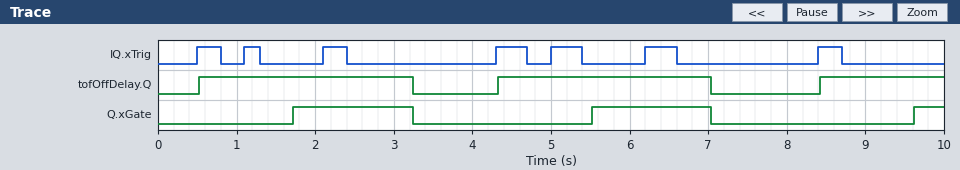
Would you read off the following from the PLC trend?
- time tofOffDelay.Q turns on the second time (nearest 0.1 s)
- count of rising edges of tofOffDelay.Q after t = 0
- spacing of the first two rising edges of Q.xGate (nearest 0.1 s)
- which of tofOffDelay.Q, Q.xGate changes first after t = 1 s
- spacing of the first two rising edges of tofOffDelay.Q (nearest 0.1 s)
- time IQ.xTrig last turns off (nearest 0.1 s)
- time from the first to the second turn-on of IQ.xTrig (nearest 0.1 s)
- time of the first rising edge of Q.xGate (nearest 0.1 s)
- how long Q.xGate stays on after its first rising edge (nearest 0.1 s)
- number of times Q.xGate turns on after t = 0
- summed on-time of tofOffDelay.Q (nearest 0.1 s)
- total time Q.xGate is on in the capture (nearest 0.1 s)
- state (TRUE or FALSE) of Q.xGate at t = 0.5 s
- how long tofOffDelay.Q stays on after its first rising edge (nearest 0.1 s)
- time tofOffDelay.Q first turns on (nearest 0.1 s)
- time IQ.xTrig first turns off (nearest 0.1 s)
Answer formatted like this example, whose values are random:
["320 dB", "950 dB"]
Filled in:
["4.3 s", "3", "3.8 s", "Q.xGate", "3.8 s", "8.7 s", "0.6 s", "1.7 s", "1.5 s", "3", "7.0 s", "3.4 s", "FALSE", "2.7 s", "0.5 s", "0.8 s"]
